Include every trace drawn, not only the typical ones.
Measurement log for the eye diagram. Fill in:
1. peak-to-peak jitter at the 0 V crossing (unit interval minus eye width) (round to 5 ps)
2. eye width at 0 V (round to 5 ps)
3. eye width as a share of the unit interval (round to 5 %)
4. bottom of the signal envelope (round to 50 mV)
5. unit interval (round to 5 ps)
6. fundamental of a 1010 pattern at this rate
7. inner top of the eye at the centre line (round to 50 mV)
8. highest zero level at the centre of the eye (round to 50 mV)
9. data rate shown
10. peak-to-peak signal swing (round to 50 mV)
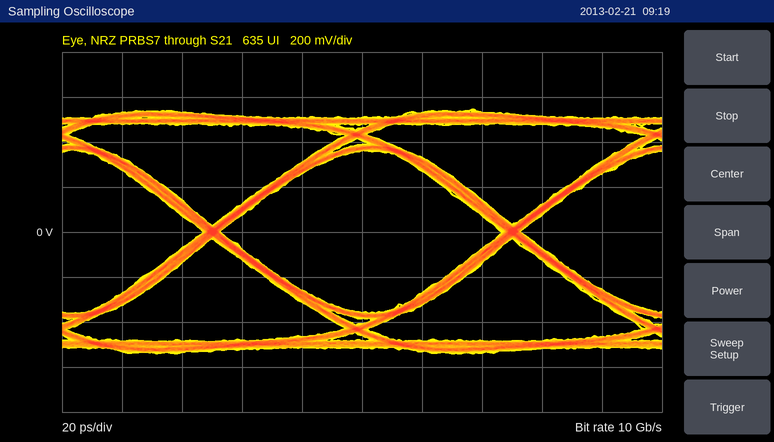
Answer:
5 ps
95 ps
95 %
-550 mV
100 ps
5 GHz
350 mV
-350 mV
10 Gb/s
1.10 V
